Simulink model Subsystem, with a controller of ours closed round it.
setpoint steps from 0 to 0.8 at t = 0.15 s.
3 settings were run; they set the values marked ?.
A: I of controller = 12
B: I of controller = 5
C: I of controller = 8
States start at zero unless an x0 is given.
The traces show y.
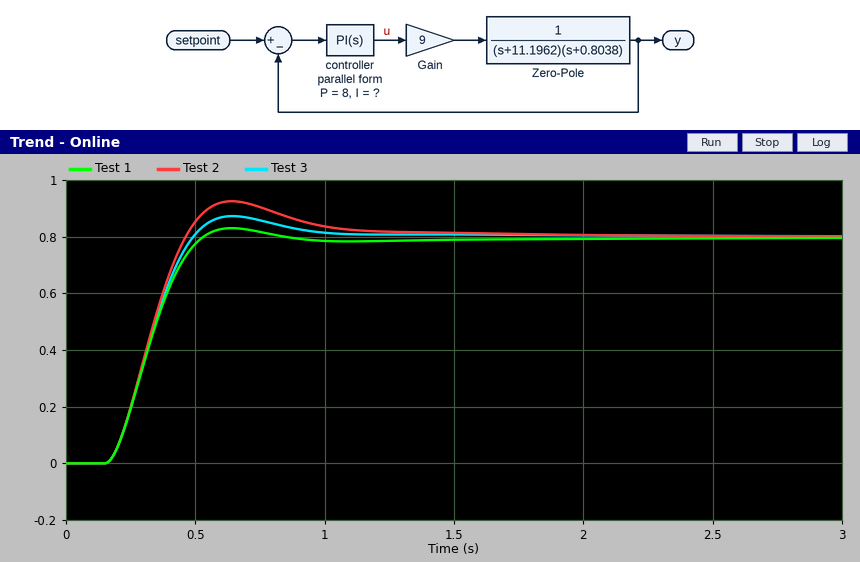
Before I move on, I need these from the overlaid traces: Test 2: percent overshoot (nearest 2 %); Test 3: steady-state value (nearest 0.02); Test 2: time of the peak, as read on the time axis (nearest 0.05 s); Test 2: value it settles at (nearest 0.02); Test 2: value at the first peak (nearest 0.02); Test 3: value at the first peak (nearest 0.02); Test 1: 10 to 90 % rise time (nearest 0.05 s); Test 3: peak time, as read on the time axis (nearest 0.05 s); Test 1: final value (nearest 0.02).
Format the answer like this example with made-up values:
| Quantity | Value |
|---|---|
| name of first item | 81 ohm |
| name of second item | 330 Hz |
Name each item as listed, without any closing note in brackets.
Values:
| Quantity | Value |
|---|---|
| Test 2: percent overshoot | 16 % |
| Test 3: steady-state value | 0.80 |
| Test 2: time of the peak, as read on the time axis | 0.65 s |
| Test 2: value it settles at | 0.80 |
| Test 2: value at the first peak | 0.92 |
| Test 3: value at the first peak | 0.88 |
| Test 1: 10 to 90 % rise time | 0.25 s |
| Test 3: peak time, as read on the time axis | 0.65 s |
| Test 1: final value | 0.80 |
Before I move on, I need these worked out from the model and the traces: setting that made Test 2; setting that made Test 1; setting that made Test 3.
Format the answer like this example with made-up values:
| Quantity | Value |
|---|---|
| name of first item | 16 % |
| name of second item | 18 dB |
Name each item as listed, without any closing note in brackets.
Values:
| Quantity | Value |
|---|---|
| setting that made Test 2 | A |
| setting that made Test 1 | B |
| setting that made Test 3 | C |
